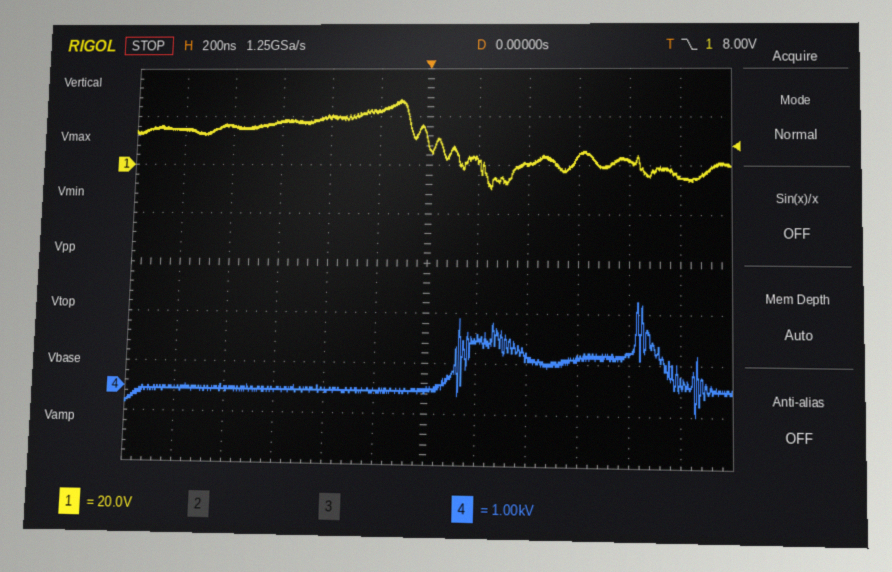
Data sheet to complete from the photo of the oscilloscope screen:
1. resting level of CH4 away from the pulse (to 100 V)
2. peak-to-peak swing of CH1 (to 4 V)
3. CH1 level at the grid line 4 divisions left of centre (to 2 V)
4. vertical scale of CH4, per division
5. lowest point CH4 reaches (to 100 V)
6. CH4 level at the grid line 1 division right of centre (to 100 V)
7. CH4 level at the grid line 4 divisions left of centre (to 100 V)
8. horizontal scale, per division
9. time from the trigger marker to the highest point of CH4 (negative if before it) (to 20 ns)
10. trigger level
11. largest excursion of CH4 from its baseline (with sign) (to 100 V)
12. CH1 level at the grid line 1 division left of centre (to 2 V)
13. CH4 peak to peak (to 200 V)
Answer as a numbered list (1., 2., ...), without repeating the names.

1. 0.0 kV
2. 36 V
3. 16 V
4. 1 kV
5. -500 V
6. 1.0 kV
7. 0.0 kV
8. 200 ns
9. +840 ns
10. 8.00 V
11. +1.8 kV
12. 22 V
13. 2.2 kV
